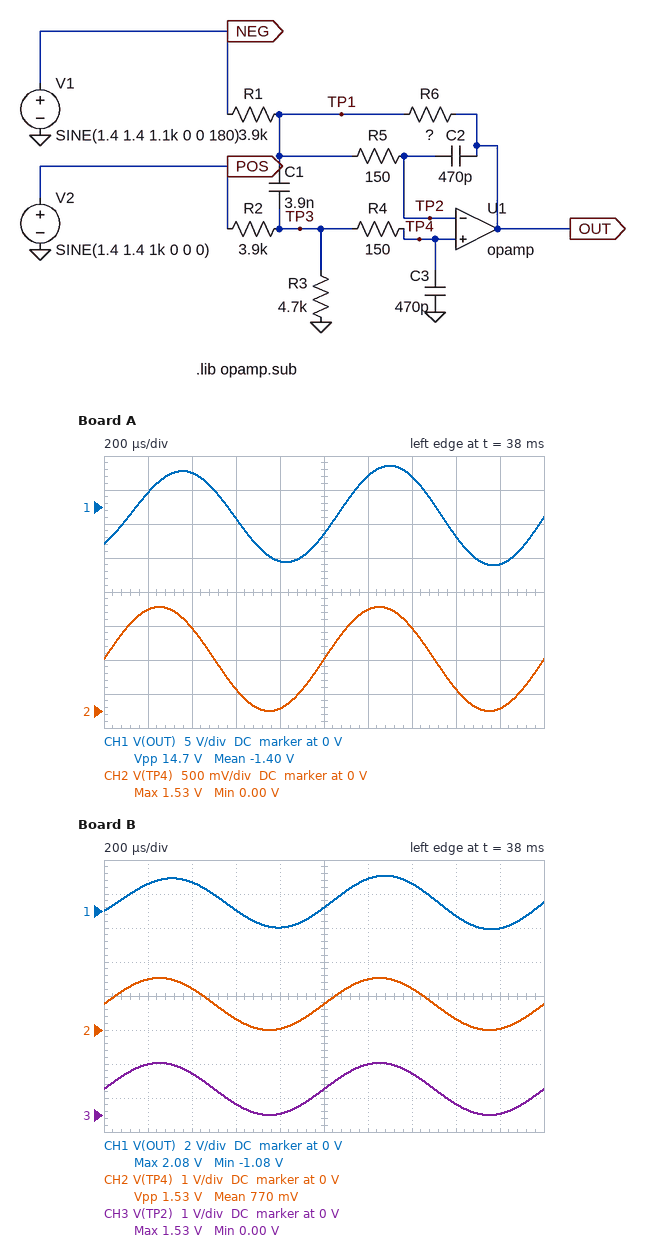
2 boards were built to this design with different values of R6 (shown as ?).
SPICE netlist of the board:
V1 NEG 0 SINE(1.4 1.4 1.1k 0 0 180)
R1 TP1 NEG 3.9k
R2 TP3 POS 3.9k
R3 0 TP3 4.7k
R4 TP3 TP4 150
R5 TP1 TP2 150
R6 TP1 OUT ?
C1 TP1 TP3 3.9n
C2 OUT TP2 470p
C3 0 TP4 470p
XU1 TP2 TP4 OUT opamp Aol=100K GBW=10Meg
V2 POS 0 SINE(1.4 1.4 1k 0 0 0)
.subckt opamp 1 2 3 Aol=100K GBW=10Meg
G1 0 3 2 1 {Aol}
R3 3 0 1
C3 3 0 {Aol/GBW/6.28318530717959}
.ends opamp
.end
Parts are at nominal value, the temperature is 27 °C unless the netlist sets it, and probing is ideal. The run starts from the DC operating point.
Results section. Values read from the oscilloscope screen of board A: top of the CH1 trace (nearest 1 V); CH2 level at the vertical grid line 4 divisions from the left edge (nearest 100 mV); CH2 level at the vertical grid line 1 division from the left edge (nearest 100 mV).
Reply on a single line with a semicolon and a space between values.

6 V; 0 V; 1.5 V
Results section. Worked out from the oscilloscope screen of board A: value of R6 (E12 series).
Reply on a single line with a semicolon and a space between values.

12 kΩ
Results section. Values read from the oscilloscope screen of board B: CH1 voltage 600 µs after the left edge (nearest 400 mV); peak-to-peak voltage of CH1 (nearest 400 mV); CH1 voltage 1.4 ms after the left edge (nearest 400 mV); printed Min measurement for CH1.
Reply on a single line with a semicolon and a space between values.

0 V; 3.2 V; 1.6 V; -1.08 V
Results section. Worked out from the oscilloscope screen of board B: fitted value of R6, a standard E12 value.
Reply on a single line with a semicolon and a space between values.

1.5 kΩ
